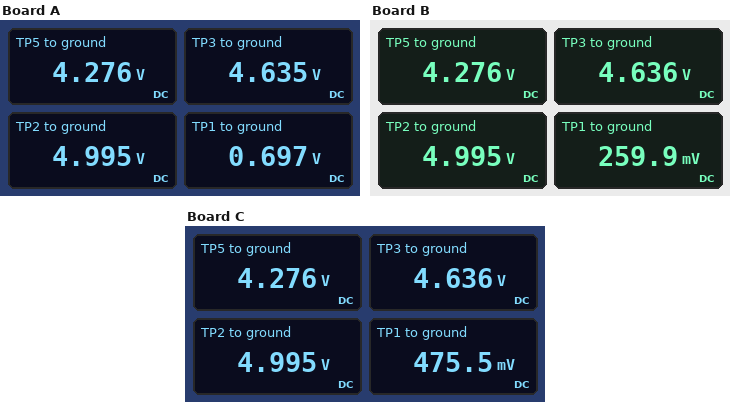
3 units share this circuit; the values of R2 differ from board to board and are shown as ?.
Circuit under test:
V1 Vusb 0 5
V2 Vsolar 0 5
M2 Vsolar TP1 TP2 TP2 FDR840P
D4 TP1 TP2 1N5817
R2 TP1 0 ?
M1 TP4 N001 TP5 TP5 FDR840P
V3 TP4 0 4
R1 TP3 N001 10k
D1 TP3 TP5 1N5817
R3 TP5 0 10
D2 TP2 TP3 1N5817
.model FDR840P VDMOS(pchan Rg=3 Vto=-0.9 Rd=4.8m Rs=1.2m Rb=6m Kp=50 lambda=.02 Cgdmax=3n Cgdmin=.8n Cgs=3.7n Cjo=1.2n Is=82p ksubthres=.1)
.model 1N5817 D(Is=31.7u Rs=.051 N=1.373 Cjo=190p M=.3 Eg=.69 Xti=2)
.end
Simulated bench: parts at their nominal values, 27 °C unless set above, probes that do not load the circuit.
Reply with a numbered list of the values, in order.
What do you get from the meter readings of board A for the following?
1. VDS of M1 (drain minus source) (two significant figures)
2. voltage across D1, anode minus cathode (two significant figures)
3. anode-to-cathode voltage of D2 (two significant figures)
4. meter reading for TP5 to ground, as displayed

1. -280 mV
2. 360 mV
3. 360 mV
4. 4.276 V
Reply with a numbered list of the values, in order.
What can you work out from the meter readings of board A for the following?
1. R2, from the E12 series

1. 22 kΩ
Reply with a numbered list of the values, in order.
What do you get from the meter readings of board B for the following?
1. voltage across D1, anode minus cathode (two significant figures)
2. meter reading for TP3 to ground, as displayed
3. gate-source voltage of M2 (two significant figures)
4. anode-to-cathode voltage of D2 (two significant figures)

1. 360 mV
2. 4.636 V
3. -4.7 V
4. 360 mV
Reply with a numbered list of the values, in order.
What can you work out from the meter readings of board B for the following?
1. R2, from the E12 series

1. 8.2 kΩ
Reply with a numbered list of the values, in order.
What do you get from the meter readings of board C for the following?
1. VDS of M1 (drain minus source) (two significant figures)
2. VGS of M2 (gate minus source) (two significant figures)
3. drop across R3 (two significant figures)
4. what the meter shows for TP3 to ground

1. -280 mV
2. -4.5 V
3. 4.3 V
4. 4.636 V
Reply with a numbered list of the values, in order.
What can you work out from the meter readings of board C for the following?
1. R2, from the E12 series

1. 15 kΩ
